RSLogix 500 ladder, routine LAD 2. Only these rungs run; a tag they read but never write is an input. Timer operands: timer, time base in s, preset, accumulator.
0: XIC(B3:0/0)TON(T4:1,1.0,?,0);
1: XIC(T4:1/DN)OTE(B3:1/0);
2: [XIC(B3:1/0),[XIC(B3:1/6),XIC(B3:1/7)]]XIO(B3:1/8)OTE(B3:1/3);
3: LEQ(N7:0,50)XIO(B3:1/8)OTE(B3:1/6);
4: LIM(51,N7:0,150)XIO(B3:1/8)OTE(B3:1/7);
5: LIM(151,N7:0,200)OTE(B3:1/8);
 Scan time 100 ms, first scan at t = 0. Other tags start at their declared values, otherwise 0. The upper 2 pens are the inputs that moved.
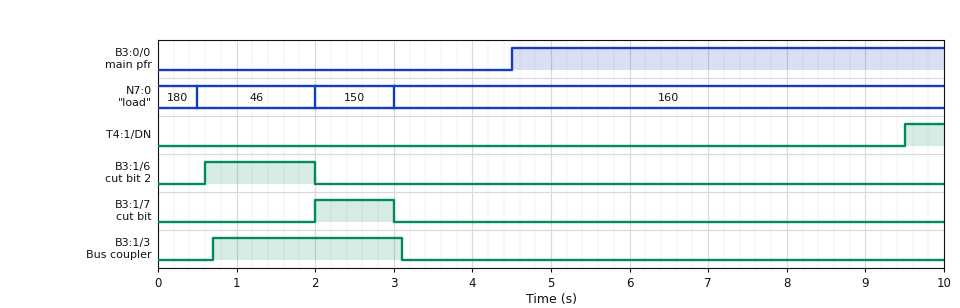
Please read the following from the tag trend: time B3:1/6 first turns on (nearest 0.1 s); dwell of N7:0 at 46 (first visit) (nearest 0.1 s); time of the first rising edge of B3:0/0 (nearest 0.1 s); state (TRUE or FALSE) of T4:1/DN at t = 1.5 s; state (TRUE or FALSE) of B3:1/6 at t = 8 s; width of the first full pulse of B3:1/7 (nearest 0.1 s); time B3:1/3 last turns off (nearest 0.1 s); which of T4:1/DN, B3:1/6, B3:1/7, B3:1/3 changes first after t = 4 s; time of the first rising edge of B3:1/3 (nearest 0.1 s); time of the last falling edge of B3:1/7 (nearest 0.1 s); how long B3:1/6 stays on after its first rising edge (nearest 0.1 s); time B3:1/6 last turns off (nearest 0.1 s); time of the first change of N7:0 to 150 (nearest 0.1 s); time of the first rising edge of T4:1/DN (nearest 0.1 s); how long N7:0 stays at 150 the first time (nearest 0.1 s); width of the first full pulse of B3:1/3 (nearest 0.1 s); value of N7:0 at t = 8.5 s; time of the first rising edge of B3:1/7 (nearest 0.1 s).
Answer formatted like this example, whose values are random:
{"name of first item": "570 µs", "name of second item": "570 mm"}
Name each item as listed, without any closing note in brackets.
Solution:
{"time B3:1/6 first turns on": "0.6 s", "dwell of N7:0 at 46 (first visit)": "1.5 s", "time of the first rising edge of B3:0/0": "4.5 s", "state (TRUE or FALSE) of T4:1/DN at t = 1.5 s": "FALSE", "state (TRUE or FALSE) of B3:1/6 at t = 8 s": "FALSE", "width of the first full pulse of B3:1/7": "1.0 s", "time B3:1/3 last turns off": "3.1 s", "which of T4:1/DN, B3:1/6, B3:1/7, B3:1/3 changes first after t = 4 s": "T4:1/DN", "time of the first rising edge of B3:1/3": "0.7 s", "time of the last falling edge of B3:1/7": "3.0 s", "how long B3:1/6 stays on after its first rising edge": "1.4 s", "time B3:1/6 last turns off": "2.0 s", "time of the first change of N7:0 to 150": "2.0 s", "time of the first rising edge of T4:1/DN": "9.5 s", "how long N7:0 stays at 150 the first time": "1.0 s", "width of the first full pulse of B3:1/3": "2.4 s", "value of N7:0 at t = 8.5 s": "160", "time of the first rising edge of B3:1/7": "2.0 s"}
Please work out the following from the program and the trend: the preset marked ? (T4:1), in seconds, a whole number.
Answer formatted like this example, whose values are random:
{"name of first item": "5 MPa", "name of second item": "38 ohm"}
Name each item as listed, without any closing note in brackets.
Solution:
{"the preset marked ? (T4:1), in seconds, a whole number": "5 s"}
